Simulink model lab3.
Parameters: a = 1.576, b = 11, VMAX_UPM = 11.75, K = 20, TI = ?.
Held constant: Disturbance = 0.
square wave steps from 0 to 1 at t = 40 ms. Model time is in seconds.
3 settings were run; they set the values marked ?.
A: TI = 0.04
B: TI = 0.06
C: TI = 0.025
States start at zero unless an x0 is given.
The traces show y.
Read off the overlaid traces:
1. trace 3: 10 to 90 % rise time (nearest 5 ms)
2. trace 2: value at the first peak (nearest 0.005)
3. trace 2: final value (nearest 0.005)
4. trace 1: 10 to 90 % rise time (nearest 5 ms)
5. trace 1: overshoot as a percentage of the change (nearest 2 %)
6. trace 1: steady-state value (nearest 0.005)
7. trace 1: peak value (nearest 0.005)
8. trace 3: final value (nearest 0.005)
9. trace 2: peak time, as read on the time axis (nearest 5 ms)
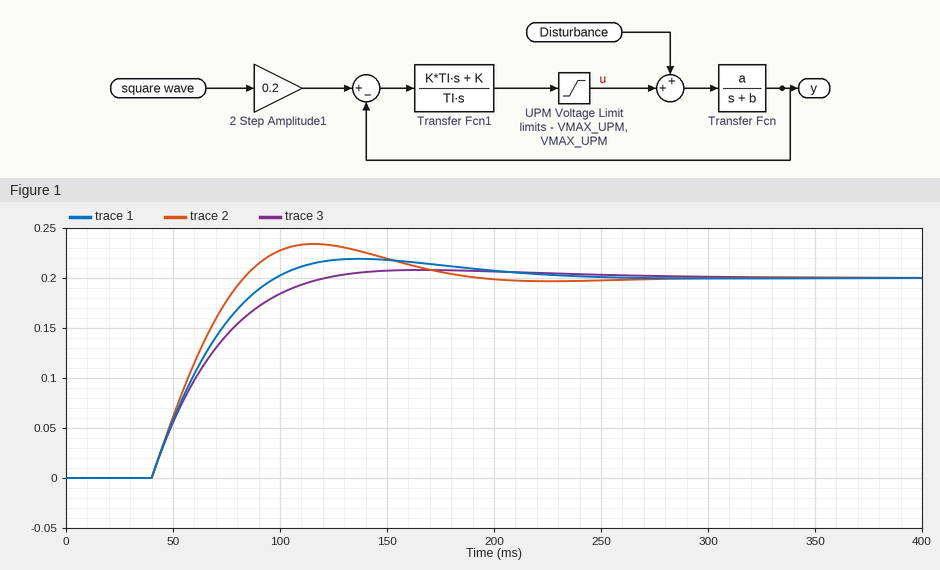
55 ms
0.235
0.200
40 ms
10 %
0.200
0.220
0.200
115 ms
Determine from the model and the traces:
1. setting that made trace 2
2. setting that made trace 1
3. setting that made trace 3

C
A
B
